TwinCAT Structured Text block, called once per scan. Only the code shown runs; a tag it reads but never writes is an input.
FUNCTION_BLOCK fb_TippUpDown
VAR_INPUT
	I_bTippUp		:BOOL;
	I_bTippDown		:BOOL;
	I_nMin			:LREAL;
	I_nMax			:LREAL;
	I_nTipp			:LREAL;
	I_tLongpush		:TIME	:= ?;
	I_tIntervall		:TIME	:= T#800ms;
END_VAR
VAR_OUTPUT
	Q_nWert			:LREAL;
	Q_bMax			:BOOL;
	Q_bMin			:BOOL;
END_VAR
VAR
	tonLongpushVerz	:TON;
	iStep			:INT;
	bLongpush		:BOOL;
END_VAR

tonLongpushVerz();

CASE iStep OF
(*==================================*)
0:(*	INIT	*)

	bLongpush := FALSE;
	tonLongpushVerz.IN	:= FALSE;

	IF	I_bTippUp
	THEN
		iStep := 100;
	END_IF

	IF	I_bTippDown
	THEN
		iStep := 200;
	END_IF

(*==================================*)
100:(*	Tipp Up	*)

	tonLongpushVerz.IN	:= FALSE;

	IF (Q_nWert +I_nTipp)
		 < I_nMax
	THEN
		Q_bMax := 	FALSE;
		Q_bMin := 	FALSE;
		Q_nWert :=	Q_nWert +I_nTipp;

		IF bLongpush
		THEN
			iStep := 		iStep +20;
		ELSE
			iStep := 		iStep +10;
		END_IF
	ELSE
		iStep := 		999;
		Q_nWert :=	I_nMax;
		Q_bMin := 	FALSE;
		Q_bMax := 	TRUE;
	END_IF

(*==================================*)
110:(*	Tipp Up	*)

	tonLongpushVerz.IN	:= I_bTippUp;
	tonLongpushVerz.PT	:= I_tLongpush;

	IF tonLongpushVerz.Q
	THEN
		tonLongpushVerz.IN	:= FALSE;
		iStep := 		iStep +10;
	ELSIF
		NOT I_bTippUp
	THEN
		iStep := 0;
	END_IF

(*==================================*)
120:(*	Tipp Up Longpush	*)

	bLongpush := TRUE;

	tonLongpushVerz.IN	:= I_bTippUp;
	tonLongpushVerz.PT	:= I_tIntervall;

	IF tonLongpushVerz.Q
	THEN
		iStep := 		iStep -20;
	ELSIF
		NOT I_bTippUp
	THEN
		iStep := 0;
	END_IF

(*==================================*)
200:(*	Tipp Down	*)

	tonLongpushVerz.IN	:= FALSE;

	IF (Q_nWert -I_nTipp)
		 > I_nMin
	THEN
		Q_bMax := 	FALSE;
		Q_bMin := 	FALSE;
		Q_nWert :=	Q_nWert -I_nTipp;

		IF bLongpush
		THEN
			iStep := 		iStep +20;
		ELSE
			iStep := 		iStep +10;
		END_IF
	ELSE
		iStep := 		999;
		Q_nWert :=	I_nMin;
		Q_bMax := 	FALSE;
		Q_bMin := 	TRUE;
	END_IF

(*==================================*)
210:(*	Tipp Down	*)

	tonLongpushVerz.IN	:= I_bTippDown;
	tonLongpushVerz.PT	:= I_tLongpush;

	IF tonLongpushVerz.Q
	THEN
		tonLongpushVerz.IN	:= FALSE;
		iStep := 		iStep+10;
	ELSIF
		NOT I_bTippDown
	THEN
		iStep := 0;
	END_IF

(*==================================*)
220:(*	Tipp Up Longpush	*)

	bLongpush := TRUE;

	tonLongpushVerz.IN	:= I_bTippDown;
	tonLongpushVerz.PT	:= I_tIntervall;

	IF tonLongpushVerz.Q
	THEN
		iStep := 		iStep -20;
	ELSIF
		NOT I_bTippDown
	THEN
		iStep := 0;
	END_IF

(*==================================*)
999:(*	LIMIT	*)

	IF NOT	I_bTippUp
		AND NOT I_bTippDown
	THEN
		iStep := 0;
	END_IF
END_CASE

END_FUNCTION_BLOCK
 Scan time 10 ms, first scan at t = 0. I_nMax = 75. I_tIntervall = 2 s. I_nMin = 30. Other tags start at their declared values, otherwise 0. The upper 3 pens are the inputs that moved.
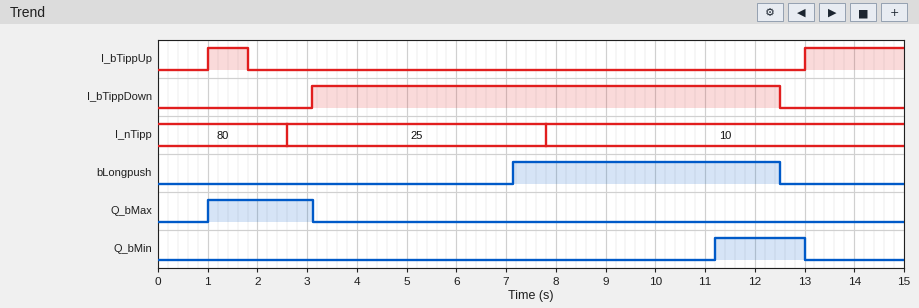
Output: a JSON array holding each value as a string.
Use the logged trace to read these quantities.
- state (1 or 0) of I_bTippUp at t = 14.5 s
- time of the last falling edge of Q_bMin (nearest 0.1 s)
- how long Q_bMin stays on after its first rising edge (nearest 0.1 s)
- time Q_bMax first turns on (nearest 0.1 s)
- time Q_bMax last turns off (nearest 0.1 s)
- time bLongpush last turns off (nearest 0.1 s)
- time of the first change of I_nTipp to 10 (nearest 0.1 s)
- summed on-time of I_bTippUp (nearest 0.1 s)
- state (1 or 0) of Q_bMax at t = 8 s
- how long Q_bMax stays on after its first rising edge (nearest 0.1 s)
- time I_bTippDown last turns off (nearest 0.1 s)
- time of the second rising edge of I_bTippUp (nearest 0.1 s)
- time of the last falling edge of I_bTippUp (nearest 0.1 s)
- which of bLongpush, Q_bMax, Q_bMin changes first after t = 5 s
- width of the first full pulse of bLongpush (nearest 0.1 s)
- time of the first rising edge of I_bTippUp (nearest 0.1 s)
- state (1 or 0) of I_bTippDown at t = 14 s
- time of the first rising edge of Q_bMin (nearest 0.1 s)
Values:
["1", "13.0 s", "1.8 s", "1.0 s", "3.1 s", "12.5 s", "7.8 s", "2.8 s", "0", "2.1 s", "12.5 s", "13.0 s", "1.8 s", "bLongpush", "5.4 s", "1.0 s", "0", "11.2 s"]
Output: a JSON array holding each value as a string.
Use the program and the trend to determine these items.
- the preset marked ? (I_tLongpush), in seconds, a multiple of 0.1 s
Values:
["4.0 s"]
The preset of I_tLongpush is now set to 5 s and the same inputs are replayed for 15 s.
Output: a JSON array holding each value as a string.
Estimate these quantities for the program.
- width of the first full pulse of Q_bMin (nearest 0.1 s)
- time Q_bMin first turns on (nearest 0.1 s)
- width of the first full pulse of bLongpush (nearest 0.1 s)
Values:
["0.8 s", "12.2 s", "4.4 s"]
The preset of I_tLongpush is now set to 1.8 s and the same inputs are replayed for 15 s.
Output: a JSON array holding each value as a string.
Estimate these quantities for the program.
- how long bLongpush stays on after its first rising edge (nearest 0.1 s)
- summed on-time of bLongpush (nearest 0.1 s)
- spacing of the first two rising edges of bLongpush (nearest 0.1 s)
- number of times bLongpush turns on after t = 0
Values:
["7.6 s", "7.7 s", "9.9 s", "2"]
